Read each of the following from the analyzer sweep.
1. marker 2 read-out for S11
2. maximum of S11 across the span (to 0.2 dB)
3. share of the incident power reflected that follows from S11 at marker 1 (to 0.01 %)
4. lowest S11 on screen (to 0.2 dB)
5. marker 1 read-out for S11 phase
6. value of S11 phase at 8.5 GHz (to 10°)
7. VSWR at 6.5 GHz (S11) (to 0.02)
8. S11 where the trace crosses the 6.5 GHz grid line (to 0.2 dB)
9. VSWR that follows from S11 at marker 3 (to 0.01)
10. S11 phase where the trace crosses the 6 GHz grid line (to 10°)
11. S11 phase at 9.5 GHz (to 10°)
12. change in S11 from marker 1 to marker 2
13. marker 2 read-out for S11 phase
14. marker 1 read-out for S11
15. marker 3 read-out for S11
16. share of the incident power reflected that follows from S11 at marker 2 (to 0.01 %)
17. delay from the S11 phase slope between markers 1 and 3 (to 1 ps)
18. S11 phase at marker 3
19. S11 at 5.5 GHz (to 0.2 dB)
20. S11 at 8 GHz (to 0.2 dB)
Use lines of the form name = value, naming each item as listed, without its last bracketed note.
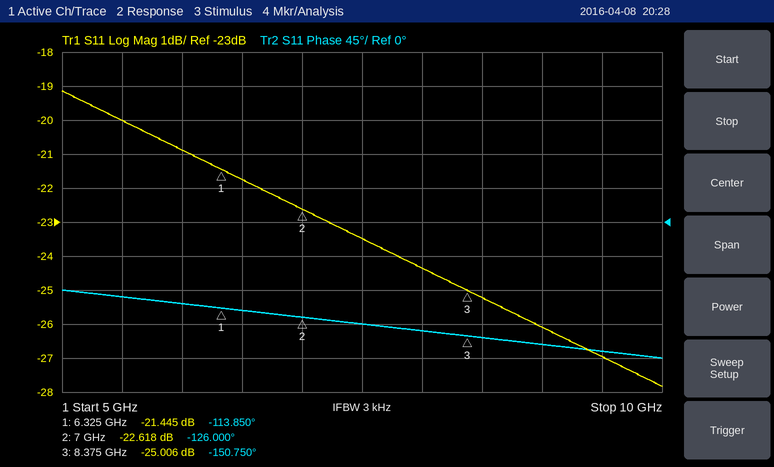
marker 2 read-out for S11 = -22.618 dB
maximum of S11 across the span = -19.2 dB
share of the incident power reflected that follows from S11 at marker 1 = 0.72 %
lowest S11 on screen = -27.8 dB
marker 1 read-out for S11 phase = -113.850°
value of S11 phase at 8.5 GHz = -150°
VSWR at 6.5 GHz (S11) = 1.18
S11 where the trace crosses the 6.5 GHz grid line = -21.8 dB
VSWR that follows from S11 at marker 3 = 1.12
S11 phase where the trace crosses the 6 GHz grid line = -110°
S11 phase at 9.5 GHz = -170°
change in S11 from marker 1 to marker 2 = -1.173 dB
marker 2 read-out for S11 phase = -126.000°
marker 1 read-out for S11 = -21.445 dB
marker 3 read-out for S11 = -25.006 dB
share of the incident power reflected that follows from S11 at marker 2 = 0.55 %
delay from the S11 phase slope between markers 1 and 3 = 50 ps
S11 phase at marker 3 = -150.750°
S11 at 5.5 GHz = -20.0 dB
S11 at 8 GHz = -24.4 dB
